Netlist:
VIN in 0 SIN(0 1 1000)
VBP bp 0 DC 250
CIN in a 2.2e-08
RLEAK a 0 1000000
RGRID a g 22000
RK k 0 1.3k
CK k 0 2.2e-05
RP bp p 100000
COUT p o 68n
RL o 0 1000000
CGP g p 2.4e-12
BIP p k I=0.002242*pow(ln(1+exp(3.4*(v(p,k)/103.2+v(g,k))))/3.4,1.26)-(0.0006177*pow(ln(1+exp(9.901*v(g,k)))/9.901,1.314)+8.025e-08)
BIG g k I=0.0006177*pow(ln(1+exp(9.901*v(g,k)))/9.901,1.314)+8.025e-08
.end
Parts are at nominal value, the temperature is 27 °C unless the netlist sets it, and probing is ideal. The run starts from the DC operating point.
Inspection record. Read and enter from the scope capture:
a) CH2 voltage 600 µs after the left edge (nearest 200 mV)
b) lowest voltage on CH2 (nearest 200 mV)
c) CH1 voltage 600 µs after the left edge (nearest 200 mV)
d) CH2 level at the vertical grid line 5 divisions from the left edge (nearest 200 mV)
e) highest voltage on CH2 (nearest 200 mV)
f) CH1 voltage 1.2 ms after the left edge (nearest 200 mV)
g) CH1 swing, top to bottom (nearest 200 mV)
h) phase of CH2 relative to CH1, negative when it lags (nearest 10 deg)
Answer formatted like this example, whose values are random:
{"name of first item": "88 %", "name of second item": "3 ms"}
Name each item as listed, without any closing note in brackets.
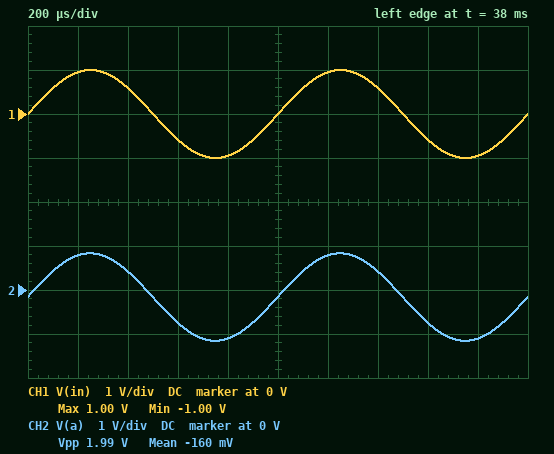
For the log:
{"CH2 voltage 600 µs after the left edge": "-800 mV", "lowest voltage on CH2": "-1.2 V", "CH1 voltage 600 µs after the left edge": "-600 mV", "CH2 level at the vertical grid line 5 divisions from the left edge": "-200 mV", "highest voltage on CH2": "800 mV", "CH1 voltage 1.2 ms after the left edge": "1.0 V", "CH1 swing, top to bottom": "2.0 V", "phase of CH2 relative to CH1, negative when it lags": "0 deg"}
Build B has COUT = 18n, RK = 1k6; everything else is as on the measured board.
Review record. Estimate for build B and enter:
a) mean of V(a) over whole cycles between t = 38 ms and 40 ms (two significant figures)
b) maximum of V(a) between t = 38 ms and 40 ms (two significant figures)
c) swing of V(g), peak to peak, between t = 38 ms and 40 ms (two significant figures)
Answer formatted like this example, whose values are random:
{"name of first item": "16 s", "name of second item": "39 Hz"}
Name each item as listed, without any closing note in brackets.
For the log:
{"mean of V(a) over whole cycles between t = 38 ms and 40 ms": "-110 mV", "maximum of V(a) between t = 38 ms and 40 ms": "890 mV", "swing of V(g), peak to peak, between t = 38 ms and 40 ms": "2.0 V"}
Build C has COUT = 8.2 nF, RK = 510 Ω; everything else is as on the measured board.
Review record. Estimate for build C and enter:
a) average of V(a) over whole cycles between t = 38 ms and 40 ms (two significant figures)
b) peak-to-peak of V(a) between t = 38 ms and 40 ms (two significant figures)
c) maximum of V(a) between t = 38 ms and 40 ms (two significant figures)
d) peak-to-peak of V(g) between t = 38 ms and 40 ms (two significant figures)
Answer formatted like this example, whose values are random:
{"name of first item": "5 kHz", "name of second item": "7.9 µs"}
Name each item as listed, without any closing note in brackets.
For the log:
{"average of V(a) over whole cycles between t = 38 ms and 40 ms": "-580 mV", "peak-to-peak of V(a) between t = 38 ms and 40 ms": "2.0 V", "maximum of V(a) between t = 38 ms and 40 ms": "420 mV", "peak-to-peak of V(g) between t = 38 ms and 40 ms": "1.9 V"}
